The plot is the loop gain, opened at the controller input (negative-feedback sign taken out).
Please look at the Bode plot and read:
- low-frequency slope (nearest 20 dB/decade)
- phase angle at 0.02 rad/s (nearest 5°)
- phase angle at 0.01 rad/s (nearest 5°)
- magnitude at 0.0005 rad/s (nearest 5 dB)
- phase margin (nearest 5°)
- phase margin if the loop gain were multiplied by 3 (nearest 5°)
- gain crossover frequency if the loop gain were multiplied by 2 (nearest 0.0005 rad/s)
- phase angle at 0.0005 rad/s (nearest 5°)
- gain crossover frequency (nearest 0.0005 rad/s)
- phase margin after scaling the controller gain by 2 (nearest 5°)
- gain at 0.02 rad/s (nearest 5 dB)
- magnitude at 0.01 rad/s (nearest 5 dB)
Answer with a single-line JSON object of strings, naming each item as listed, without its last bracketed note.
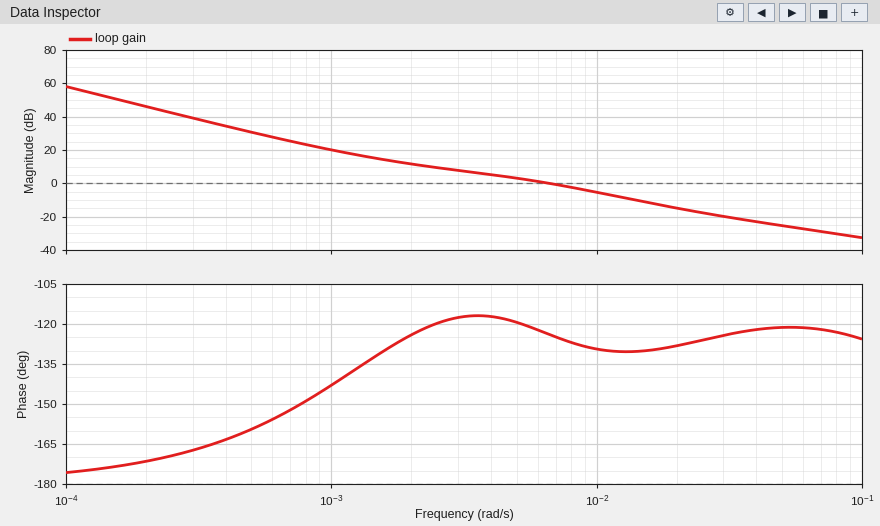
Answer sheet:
{"low-frequency slope": "-40 dB/decade", "phase angle at 0.02 rad/s": "-130°", "phase angle at 0.01 rad/s": "-130°", "magnitude at 0.0005 rad/s": "30 dB", "phase margin": "55°", "phase margin if the loop gain were multiplied by 3": "50°", "gain crossover frequency if the loop gain were multiplied by 2": "0.0105 rad/s", "phase angle at 0.0005 rad/s": "-160°", "gain crossover frequency": "0.0065 rad/s", "phase margin after scaling the controller gain by 2": "50°", "gain at 0.02 rad/s": "-15 dB", "magnitude at 0.01 rad/s": "-5 dB"}
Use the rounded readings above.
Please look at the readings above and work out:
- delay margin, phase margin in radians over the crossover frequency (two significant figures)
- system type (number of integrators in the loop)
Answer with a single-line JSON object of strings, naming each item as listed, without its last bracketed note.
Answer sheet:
{"delay margin, phase margin in radians over the crossover frequency": "150 s", "system type": "2"}
